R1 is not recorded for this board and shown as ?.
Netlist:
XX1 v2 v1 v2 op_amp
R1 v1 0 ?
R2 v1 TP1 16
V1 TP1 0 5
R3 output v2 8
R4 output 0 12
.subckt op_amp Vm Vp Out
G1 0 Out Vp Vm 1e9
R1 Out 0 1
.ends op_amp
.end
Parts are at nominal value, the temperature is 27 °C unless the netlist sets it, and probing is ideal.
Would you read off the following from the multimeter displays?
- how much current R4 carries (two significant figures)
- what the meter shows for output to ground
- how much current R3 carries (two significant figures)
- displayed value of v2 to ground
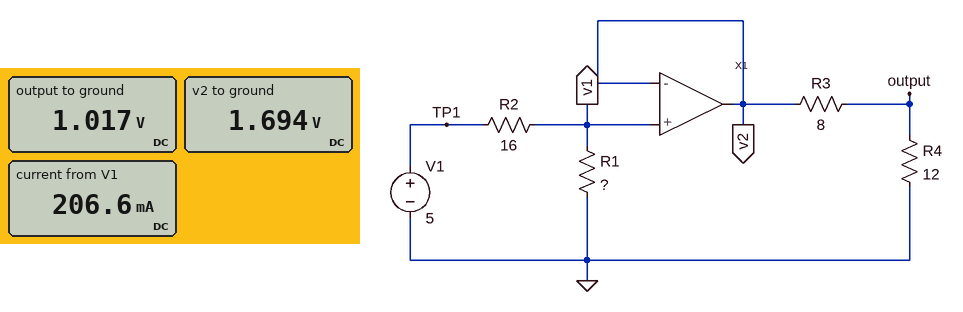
85 mA
1.017 V
85 mA
1.694 V
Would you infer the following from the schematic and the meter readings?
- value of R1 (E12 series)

8.2 Ω
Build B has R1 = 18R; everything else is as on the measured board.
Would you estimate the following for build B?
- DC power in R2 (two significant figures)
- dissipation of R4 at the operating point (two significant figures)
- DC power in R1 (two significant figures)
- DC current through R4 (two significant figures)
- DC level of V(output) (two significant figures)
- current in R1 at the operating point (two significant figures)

350 mW
210 mW
390 mW
130 mA
1.6 V
150 mA
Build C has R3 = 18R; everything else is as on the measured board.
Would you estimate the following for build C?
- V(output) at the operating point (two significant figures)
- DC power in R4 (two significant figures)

680 mV
38 mW
